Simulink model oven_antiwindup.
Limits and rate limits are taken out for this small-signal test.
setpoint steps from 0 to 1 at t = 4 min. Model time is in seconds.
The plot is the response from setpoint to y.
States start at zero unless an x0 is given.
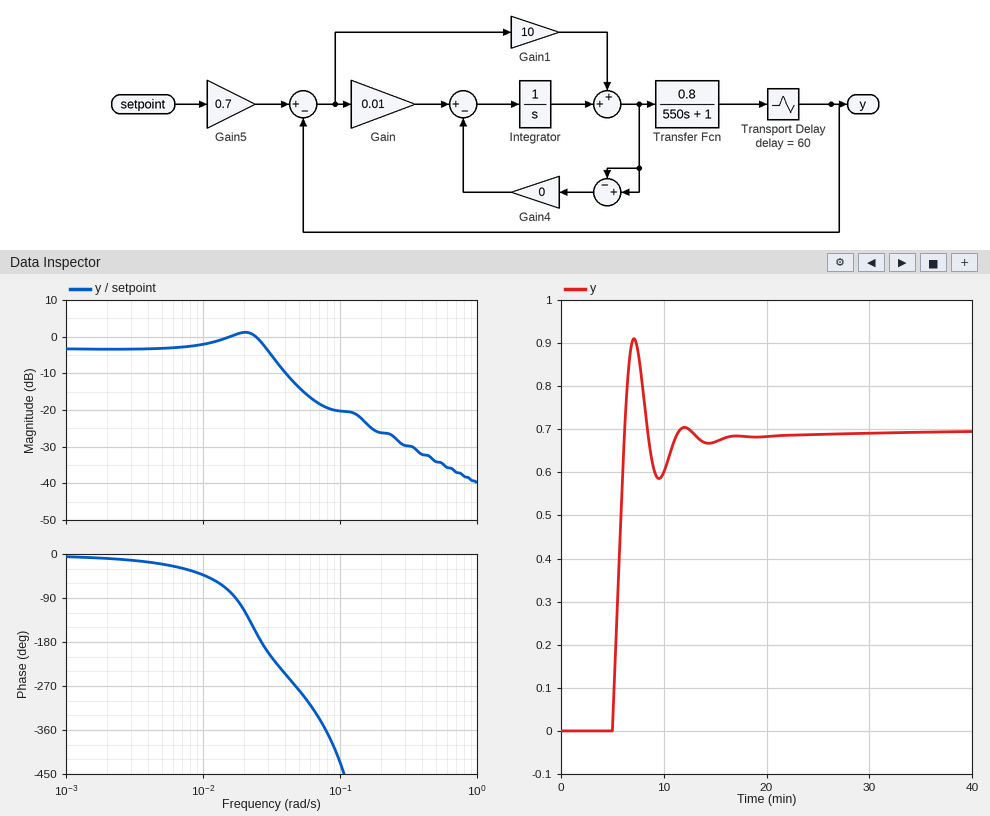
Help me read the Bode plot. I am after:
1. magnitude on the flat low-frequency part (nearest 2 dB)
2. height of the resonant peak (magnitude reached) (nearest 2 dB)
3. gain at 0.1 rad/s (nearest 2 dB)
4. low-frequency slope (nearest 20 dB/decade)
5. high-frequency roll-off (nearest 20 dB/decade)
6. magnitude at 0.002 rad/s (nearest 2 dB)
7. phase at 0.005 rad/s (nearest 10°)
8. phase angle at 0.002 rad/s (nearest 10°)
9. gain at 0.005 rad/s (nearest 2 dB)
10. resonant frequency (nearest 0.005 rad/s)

-4 dB
2 dB
-20 dB
0 dB/decade
-20 dB/decade
-4 dB
-20°
-10°
-4 dB
0.020 rad/s
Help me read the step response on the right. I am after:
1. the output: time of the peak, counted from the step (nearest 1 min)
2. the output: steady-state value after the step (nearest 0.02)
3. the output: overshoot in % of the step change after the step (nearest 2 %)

3 min
0.70
30 %
